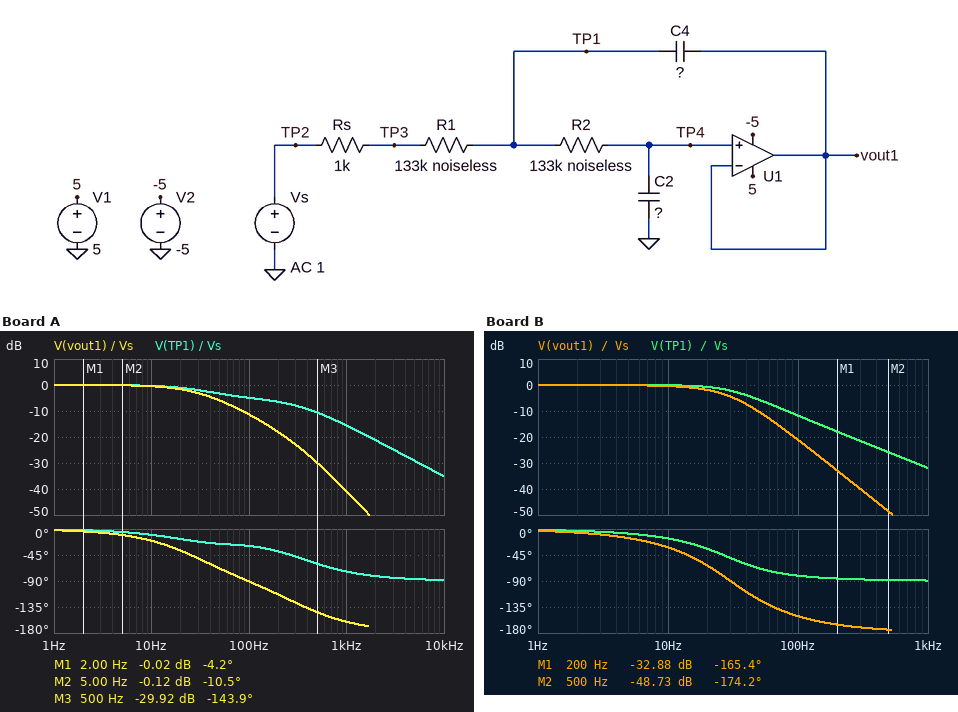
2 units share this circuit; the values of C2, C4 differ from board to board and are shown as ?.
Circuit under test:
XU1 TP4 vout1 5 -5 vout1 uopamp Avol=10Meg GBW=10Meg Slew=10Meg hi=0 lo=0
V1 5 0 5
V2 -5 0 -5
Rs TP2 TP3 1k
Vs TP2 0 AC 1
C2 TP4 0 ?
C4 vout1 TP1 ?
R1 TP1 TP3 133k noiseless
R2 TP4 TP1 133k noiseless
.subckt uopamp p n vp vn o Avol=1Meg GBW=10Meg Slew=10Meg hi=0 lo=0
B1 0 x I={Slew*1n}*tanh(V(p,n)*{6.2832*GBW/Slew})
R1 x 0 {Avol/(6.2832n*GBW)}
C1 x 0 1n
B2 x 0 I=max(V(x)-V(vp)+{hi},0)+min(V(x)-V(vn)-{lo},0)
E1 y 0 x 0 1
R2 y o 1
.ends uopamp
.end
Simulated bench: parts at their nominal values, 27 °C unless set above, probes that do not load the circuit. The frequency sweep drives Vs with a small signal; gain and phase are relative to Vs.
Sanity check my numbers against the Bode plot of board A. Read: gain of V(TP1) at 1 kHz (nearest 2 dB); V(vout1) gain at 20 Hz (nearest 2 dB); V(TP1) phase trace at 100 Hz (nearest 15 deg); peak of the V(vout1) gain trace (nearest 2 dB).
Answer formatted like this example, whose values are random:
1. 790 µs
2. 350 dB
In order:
1. -16 dB
2. -2 dB
3. -30 deg
4. 0 dB
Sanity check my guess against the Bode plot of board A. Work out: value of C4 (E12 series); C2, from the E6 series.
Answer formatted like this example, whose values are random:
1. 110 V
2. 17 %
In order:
1. 6.8 nF
2. 22 nF
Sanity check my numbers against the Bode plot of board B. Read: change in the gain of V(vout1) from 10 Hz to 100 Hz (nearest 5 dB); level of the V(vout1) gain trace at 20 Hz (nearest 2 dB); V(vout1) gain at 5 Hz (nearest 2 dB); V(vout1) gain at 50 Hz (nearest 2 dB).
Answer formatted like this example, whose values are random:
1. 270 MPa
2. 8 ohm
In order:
1. -20 dB
2. -2 dB
3. 0 dB
4. -10 dB
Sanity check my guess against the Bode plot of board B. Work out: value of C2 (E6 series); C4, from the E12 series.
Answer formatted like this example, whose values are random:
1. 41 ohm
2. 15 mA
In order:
1. 33 nF
2. 47 nF
